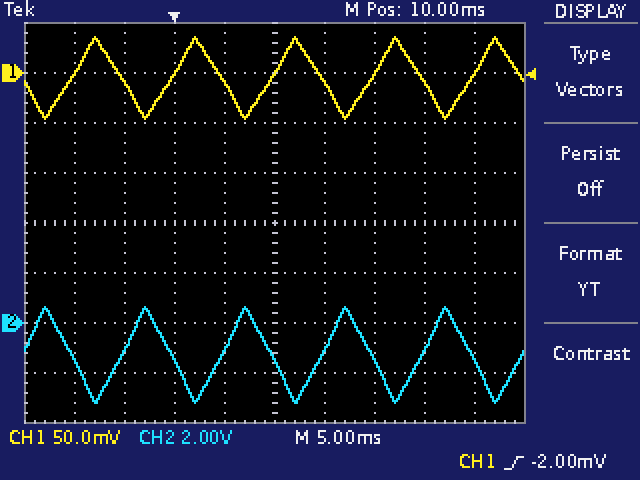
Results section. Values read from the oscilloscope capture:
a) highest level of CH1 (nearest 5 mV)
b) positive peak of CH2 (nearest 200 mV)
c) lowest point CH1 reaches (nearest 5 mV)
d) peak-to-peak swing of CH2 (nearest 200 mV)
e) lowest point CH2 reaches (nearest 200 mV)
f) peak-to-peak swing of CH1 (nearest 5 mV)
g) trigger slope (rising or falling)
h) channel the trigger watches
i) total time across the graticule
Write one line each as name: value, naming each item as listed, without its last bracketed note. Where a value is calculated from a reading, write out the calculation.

highest level of CH1: 35 mV
positive peak of CH2: 600 mV
lowest point CH1 reaches: -45 mV
peak-to-peak swing of CH2: 600 mV − (-3.2 V) = 3.8 V
lowest point CH2 reaches: -3.2 V
peak-to-peak swing of CH1: 35 mV − (-45 mV) = 80 mV
trigger slope: rising
channel the trigger watches: CH1
total time across the graticule: 50 ms
